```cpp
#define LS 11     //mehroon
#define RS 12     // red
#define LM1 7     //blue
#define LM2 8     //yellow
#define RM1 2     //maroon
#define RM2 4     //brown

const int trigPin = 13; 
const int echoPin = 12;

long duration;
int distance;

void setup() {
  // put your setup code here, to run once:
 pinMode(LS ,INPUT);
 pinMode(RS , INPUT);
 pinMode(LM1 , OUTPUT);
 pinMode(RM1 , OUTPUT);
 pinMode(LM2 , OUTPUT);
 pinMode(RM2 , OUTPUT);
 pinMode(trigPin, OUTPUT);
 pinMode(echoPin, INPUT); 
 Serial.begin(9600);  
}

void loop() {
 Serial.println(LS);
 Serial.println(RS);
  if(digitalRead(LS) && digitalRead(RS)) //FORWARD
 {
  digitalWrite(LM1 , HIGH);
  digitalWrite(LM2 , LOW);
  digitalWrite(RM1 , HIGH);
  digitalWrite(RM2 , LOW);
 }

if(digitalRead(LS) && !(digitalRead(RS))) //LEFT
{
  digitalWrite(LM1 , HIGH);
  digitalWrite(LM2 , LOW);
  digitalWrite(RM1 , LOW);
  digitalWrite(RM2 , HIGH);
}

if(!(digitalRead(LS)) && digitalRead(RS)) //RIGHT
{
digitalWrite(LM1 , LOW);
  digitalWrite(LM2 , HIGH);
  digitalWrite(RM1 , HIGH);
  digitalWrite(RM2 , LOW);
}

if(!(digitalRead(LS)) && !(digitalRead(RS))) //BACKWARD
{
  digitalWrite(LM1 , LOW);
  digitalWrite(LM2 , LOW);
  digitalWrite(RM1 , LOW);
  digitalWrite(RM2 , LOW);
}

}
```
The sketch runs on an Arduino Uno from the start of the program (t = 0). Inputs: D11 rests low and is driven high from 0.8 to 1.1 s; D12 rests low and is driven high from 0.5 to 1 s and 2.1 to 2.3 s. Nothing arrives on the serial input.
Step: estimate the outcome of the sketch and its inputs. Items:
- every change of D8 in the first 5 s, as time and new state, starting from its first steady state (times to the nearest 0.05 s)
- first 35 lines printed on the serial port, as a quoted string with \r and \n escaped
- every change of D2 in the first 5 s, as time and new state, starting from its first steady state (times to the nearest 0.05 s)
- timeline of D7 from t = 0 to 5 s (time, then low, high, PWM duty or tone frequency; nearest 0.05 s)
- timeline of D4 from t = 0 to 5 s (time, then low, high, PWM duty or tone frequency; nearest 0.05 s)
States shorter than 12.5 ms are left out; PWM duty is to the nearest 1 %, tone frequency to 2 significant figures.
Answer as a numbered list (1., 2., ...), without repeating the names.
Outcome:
1. 0 s low; 0.5 s high; 0.8 s low; 2.1 s high; 2.3 s low
2. "11\r\n12\r\n11\r\n12\r\n11\r\n12\r\n11\r\n12\r\n11\r\n12\r\n11\r\n12\r\n11\r\n12\r\n11\r\n12\r\n11\r\n12\r\n11\r\n12\r\n11\r\n12\r\n11\r\n12\r\n11\r\n12\r\n11\r\n12\r\n11\r\n12\r\n11\r\n12\r\n11\r\n12\r\n11\r\n"
3. 0 s low; 0.5 s high; 1 s low; 2.1 s high; 2.3 s low
4. 0 s low; 0.8 s high; 1.1 s low
5. 0 s low; 1 s high; 1.1 s low
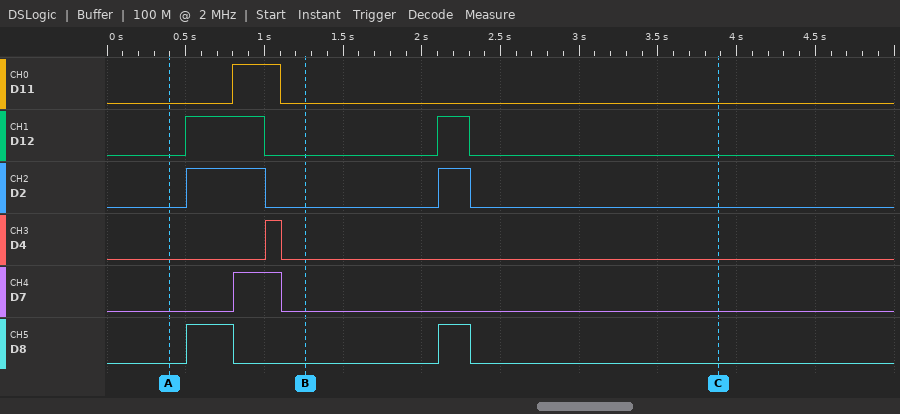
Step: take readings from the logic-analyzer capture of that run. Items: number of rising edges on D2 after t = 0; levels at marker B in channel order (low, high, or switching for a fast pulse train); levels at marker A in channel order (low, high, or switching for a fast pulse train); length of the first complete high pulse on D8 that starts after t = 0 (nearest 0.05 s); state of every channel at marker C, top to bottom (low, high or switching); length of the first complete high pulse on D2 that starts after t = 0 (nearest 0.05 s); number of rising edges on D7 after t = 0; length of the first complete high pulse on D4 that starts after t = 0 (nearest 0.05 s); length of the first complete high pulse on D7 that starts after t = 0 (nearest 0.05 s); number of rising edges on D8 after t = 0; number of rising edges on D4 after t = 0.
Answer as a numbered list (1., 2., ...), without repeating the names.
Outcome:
1. 2
2. D11 low, D12 low, D2 low, D4 low, D7 low, D8 low
3. D11 low, D12 low, D2 low, D4 low, D7 low, D8 low
4. 0.30 s
5. D11 low, D12 low, D2 low, D4 low, D7 low, D8 low
6. 0.50 s
7. 1
8. 0.10 s
9. 0.30 s
10. 2
11. 1
